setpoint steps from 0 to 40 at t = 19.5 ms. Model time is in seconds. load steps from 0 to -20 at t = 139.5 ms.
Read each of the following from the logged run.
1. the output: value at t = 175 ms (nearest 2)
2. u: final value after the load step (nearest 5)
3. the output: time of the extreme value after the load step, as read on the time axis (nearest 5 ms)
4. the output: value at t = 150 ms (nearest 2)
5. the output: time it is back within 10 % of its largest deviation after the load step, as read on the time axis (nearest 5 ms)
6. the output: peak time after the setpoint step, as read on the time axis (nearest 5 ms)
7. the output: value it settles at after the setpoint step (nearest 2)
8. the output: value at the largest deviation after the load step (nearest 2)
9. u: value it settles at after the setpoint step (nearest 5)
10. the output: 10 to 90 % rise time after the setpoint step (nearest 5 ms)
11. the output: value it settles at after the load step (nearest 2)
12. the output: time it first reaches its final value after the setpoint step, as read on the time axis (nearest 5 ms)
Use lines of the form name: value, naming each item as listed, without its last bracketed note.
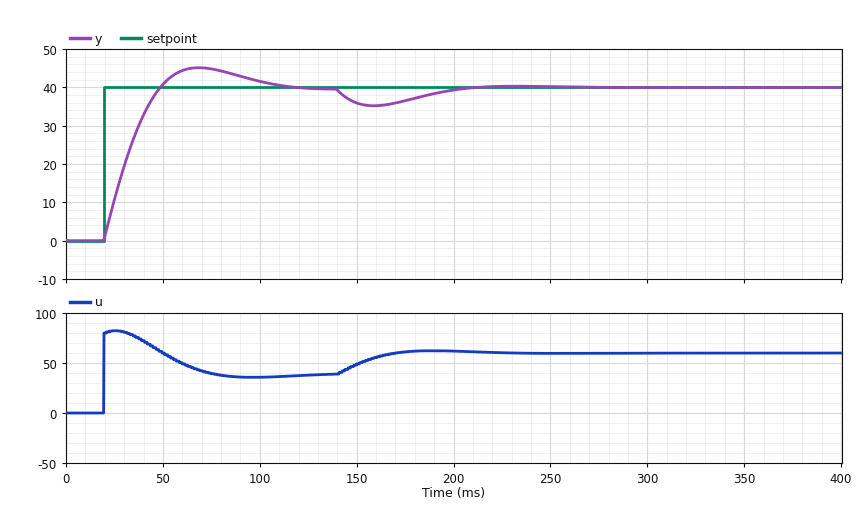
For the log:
the output: value at t = 175 ms: 36
u: final value after the load step: 60
the output: time of the extreme value after the load step, as read on the time axis: 160 ms
the output: value at t = 150 ms: 36
the output: time it is back within 10 % of its largest deviation after the load step, as read on the time axis: 205 ms
the output: peak time after the setpoint step, as read on the time axis: 70 ms
the output: value it settles at after the setpoint step: 40
the output: value at the largest deviation after the load step: 36
u: value it settles at after the setpoint step: 40
the output: 10 to 90 % rise time after the setpoint step: 20 ms
the output: value it settles at after the load step: 40
the output: time it first reaches its final value after the setpoint step, as read on the time axis: 50 ms
